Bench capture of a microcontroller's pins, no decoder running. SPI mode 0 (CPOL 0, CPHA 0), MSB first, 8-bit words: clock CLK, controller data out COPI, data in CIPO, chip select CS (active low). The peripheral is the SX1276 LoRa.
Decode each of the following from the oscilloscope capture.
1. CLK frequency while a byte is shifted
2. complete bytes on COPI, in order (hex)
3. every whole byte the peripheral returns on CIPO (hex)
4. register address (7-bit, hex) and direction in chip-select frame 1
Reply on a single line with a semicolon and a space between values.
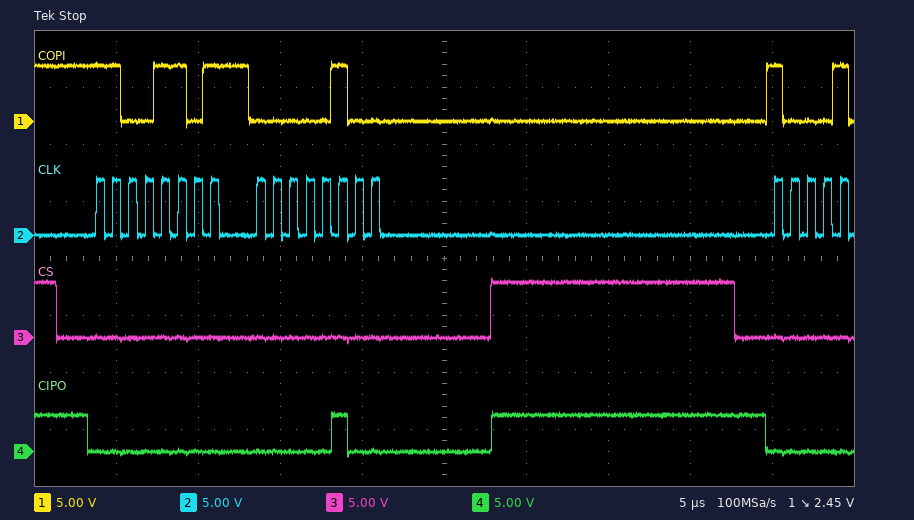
1 MHz; CD 04; 00 04; 0x4D write
